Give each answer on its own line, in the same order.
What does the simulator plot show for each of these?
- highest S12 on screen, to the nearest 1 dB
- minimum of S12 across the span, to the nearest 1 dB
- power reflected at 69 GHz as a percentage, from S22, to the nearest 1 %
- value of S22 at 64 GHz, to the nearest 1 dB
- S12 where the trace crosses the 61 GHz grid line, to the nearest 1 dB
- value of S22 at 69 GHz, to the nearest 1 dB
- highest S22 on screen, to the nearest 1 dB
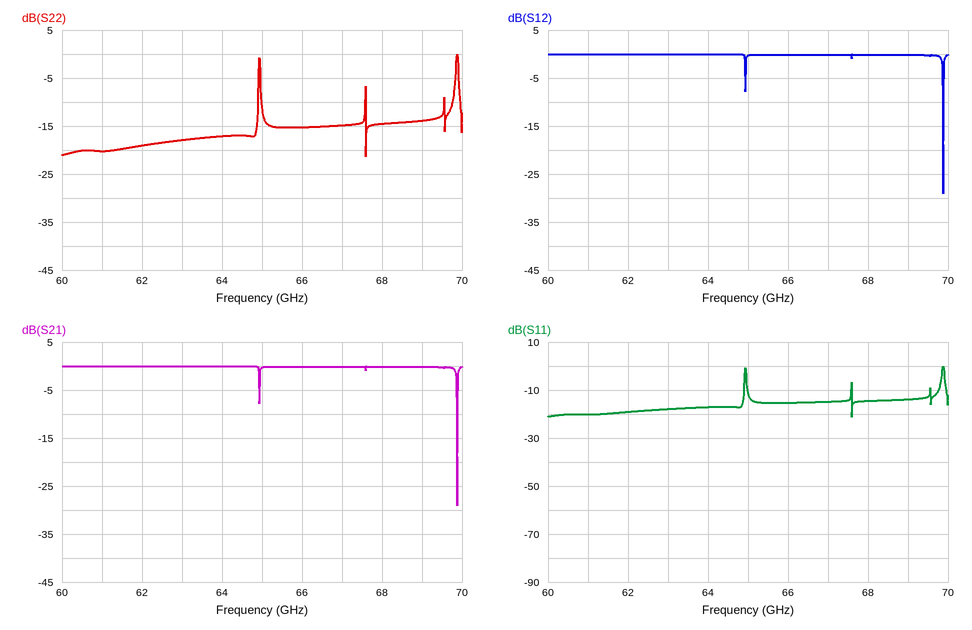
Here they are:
0 dB
-29 dB
4 %
-17 dB
0 dB
-14 dB
0 dB
